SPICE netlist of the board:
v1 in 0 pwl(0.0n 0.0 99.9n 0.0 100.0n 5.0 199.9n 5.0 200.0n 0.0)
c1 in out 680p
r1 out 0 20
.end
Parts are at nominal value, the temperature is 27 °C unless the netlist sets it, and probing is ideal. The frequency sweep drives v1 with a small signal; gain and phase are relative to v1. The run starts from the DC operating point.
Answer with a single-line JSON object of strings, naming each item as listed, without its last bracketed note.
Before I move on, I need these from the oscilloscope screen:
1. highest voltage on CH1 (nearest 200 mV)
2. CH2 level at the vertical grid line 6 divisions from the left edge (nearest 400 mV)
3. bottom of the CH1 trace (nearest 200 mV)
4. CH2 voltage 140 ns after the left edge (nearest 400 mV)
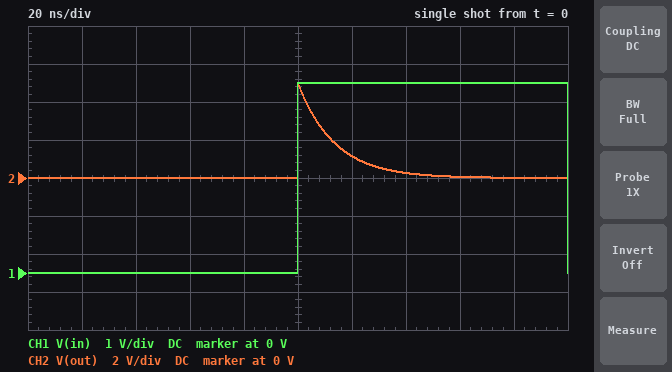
{"highest voltage on CH1": "5.0 V", "CH2 level at the vertical grid line 6 divisions from the left edge": "1.2 V", "bottom of the CH1 trace": "0 V", "CH2 voltage 140 ns after the left edge": "400 mV"}
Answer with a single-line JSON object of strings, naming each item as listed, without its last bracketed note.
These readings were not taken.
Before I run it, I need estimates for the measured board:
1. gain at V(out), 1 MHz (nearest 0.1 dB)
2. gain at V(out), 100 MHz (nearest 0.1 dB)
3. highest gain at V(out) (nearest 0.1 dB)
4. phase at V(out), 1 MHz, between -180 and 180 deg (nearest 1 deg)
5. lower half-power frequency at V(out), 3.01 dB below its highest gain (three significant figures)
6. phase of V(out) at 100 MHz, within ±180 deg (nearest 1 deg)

{"gain at V(out), 1 MHz": "-21.4 dB", "gain at V(out), 100 MHz": "-0.1 dB", "highest gain at V(out)": "0 dB", "phase at V(out), 1 MHz, between -180 and 180 deg": "85 deg", "lower half-power frequency at V(out), 3.01 dB below its highest gain": "11.7 MHz", "phase of V(out) at 100 MHz, within ±180 deg": "7 deg"}
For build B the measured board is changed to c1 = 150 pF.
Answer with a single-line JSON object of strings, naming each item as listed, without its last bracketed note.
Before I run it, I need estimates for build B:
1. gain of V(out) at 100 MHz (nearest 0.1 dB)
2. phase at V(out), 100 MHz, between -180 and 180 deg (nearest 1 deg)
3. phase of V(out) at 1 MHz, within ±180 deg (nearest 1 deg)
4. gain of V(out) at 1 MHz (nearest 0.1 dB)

{"gain of V(out) at 100 MHz": "-1.1 dB", "phase at V(out), 100 MHz, between -180 and 180 deg": "28 deg", "phase of V(out) at 1 MHz, within ±180 deg": "89 deg", "gain of V(out) at 1 MHz": "-34.5 dB"}
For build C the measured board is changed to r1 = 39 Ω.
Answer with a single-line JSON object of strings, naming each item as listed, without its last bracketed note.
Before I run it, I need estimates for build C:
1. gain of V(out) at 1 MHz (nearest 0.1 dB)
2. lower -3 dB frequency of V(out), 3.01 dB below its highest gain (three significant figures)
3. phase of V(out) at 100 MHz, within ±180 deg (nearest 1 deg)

{"gain of V(out) at 1 MHz": "-15.7 dB", "lower -3 dB frequency of V(out), 3.01 dB below its highest gain": "6.00 MHz", "phase of V(out) at 100 MHz, within ±180 deg": "3 deg"}
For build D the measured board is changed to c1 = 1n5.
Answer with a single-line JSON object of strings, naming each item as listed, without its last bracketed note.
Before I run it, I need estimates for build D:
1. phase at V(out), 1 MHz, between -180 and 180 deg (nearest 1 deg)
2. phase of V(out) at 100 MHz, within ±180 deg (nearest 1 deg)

{"phase at V(out), 1 MHz, between -180 and 180 deg": "79 deg", "phase of V(out) at 100 MHz, within ±180 deg": "3 deg"}
